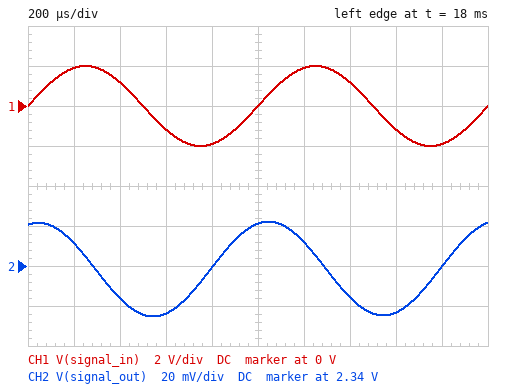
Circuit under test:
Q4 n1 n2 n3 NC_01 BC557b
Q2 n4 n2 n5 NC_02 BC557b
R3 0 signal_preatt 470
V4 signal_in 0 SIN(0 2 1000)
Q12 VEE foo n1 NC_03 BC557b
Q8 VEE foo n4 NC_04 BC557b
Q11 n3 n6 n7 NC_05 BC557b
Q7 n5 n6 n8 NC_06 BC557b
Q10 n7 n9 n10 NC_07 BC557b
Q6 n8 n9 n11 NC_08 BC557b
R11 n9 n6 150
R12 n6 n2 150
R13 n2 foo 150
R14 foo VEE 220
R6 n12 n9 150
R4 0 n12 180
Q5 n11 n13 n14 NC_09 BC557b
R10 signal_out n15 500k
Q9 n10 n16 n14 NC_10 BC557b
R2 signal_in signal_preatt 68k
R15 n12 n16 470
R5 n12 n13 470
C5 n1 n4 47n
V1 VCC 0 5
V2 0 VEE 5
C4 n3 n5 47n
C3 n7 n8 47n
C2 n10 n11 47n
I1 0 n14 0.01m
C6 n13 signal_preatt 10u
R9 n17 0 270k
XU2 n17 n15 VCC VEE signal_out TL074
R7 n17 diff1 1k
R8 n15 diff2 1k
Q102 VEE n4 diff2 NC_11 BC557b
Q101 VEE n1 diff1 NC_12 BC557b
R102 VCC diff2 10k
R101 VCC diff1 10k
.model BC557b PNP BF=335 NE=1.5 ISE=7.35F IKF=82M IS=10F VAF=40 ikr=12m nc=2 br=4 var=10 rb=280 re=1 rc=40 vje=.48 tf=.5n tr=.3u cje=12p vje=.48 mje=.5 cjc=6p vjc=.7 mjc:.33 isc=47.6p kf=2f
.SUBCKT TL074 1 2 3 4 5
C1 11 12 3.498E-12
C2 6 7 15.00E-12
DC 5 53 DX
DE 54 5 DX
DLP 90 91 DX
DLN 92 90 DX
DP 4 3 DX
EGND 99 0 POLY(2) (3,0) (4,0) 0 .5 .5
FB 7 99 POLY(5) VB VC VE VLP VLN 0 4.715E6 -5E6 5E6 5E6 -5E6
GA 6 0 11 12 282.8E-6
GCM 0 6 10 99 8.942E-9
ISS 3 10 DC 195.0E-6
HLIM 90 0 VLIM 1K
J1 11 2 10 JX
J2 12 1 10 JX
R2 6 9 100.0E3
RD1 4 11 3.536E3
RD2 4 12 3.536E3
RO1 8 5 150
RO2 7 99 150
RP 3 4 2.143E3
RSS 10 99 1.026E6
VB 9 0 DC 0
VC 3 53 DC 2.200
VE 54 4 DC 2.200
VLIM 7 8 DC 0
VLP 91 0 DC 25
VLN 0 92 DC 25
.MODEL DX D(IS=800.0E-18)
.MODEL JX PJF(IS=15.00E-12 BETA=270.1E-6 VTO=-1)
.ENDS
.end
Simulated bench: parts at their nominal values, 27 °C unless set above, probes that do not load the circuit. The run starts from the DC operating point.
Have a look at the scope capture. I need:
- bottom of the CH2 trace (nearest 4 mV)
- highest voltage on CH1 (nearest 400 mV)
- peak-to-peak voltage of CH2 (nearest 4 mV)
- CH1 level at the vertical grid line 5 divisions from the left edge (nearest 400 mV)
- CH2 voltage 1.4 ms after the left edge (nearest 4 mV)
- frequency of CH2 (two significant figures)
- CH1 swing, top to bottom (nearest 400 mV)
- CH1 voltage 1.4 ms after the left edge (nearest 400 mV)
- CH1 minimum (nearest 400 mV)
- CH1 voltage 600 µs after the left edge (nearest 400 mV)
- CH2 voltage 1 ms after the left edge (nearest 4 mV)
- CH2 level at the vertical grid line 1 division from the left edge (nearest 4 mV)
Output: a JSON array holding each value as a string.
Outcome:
["2.316 V", "2.0 V", "48 mV", "0 V", "2.324 V", "1.0 kHz", "4.0 V", "1.2 V", "-2.0 V", "-1.2 V", "2.360 V", "2.352 V"]
